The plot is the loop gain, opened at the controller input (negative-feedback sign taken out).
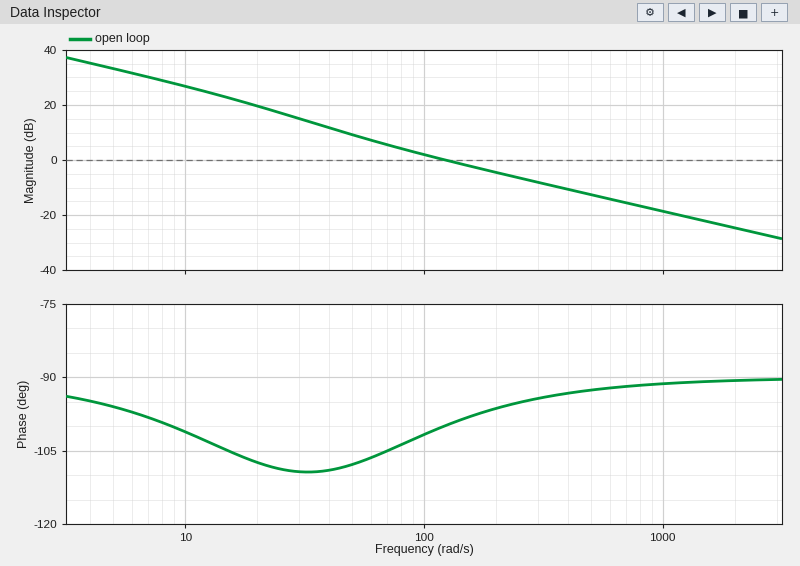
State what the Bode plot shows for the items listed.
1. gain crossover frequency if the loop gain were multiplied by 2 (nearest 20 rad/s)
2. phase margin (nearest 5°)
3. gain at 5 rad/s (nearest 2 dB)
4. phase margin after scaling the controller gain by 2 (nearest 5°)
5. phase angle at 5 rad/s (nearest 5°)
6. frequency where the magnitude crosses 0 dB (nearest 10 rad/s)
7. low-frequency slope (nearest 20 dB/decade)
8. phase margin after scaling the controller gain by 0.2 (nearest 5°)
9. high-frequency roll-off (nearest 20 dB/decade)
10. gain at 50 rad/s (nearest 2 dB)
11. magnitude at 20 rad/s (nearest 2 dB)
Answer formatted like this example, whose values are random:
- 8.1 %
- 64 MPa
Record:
- 240 rad/s
- 80°
- 34 dB
- 85°
- -95°
- 120 rad/s
- -20 dB/decade
- 70°
- -20 dB/decade
- 10 dB
- 20 dB
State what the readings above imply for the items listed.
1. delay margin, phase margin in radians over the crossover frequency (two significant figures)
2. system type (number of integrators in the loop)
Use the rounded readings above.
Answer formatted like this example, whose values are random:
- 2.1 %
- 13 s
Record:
- 0.012 s
- 1
